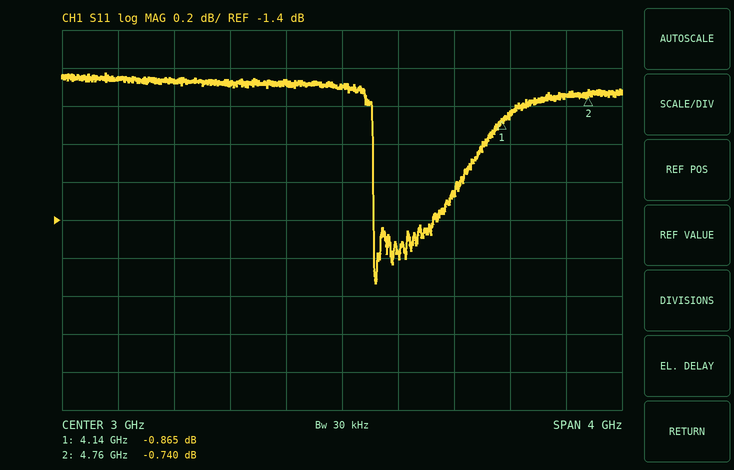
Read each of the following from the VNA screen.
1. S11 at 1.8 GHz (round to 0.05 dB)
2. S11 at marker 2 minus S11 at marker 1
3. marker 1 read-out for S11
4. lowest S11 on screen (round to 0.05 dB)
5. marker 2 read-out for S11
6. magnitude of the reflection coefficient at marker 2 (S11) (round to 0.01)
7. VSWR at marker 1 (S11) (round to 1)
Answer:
-0.65 dB
0.125 dB
-0.865 dB
-1.75 dB
-0.740 dB
0.92
20
